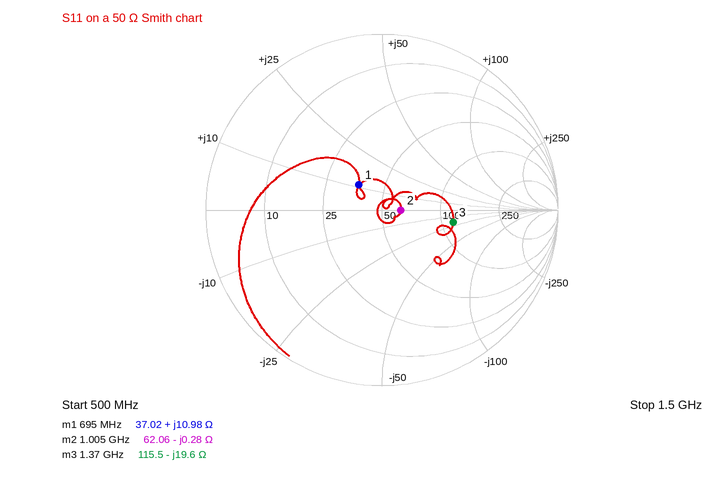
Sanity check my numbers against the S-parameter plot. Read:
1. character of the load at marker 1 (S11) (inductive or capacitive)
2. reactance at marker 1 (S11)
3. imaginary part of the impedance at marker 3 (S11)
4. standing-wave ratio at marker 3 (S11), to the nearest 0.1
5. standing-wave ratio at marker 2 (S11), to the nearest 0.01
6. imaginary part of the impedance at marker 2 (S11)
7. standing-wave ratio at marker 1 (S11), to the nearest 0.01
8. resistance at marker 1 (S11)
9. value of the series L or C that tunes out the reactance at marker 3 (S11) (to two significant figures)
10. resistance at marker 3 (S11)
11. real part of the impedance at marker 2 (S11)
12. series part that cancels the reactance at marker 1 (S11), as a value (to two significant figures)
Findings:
inductive
+10.98 Ω
-19.6 Ω
2.4
1.24
-0.28 Ω
1.48
37.02 Ω
2.3 nH
115.5 Ω
62.06 Ω
21 pF
